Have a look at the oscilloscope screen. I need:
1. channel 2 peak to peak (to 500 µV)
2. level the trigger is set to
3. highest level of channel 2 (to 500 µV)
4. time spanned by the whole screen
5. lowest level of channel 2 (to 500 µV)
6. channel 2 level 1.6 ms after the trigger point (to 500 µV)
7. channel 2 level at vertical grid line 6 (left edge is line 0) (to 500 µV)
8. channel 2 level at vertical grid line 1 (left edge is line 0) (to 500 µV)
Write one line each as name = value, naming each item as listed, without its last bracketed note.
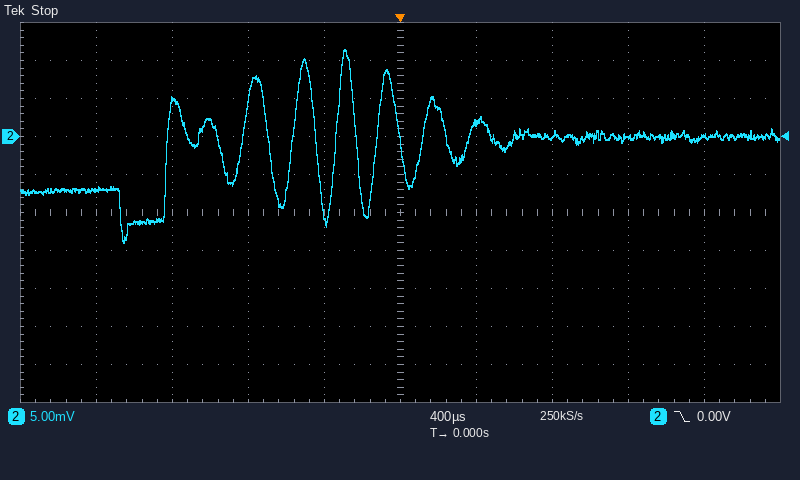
channel 2 peak to peak = 25.5 mV
level the trigger is set to = 0.00 V
highest level of channel 2 = 11.5 mV
time spanned by the whole screen = 4 ms
lowest level of channel 2 = -14.0 mV
channel 2 level 1.6 ms after the trigger point = 0.0 mV
channel 2 level at vertical grid line 6 (left edge is line 0) = 2.0 mV
channel 2 level at vertical grid line 1 (left edge is line 0) = -7.0 mV
